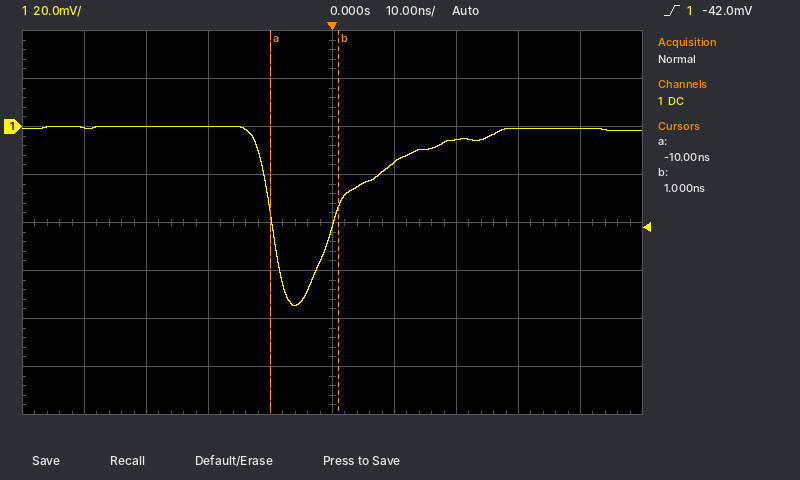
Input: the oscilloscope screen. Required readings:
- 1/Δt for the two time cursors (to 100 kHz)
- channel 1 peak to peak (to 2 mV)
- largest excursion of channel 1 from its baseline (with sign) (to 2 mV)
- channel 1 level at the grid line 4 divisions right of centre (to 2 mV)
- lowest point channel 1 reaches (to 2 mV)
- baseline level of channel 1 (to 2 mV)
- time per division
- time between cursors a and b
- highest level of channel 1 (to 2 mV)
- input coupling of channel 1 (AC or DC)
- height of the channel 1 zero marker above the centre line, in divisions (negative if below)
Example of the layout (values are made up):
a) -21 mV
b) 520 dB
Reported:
a) 90.9 MHz
b) 74 mV
c) -74 mV
d) 0 mV
e) -74 mV
f) 0 mV
g) 10 ns
h) 11 ns
i) 0 mV
j) DC
k) +2.0 div
